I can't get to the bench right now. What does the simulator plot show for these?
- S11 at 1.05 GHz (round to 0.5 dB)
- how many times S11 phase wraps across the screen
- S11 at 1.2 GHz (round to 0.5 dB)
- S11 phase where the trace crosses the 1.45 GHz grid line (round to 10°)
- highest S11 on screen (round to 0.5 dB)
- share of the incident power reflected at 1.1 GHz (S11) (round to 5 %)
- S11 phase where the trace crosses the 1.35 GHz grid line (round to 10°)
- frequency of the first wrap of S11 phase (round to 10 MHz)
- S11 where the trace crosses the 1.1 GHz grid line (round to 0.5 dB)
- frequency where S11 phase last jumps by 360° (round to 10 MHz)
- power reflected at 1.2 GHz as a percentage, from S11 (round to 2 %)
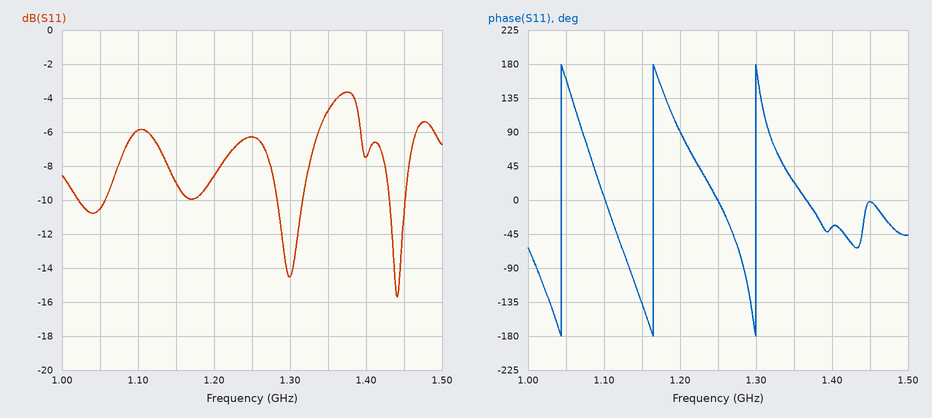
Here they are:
-10.5 dB
3
-8.5 dB
0°
-3.5 dB
25 %
20°
1.04 GHz
-6.0 dB
1.30 GHz
14 %
